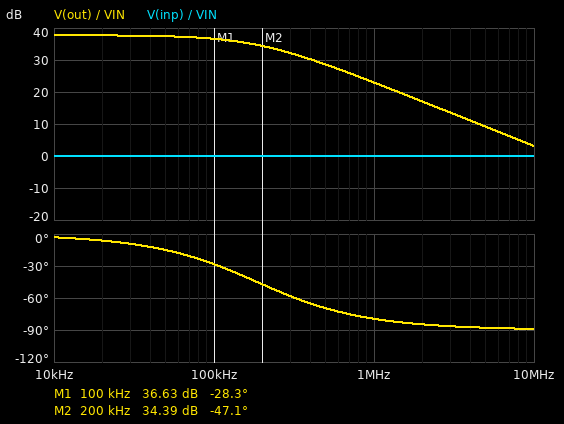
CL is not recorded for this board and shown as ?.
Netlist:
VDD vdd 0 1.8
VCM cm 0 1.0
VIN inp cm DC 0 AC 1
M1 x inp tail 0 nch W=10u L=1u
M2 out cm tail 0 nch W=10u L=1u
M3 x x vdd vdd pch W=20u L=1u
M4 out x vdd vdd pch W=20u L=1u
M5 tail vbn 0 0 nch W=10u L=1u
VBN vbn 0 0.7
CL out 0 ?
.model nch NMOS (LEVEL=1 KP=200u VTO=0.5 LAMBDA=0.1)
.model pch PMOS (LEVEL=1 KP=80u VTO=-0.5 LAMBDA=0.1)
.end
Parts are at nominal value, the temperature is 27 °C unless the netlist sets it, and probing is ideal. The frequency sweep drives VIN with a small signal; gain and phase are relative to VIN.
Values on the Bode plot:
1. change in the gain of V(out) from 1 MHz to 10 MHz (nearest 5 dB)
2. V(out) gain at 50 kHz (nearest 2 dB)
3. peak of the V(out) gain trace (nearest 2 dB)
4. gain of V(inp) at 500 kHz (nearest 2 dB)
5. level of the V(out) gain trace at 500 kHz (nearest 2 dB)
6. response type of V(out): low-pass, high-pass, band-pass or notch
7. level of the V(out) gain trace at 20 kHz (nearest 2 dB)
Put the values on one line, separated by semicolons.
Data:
-20 dB; 38 dB; 38 dB; 0 dB; 28 dB; low-pass; 38 dB
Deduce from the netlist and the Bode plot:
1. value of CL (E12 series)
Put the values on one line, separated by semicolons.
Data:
3.3 pF
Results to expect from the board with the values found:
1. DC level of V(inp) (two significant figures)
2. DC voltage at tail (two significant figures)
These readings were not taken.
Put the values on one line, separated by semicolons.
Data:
1.0 V; 360 mV
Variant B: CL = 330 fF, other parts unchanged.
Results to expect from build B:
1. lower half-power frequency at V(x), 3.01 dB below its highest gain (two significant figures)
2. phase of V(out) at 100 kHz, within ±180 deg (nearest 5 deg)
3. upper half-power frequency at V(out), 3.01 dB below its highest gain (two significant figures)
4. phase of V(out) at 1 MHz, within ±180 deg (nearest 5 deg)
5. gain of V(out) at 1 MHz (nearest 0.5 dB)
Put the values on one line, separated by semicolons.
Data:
1.3 MHz; -5 deg; 1.9 MHz; -30 deg; 36.5 dB
